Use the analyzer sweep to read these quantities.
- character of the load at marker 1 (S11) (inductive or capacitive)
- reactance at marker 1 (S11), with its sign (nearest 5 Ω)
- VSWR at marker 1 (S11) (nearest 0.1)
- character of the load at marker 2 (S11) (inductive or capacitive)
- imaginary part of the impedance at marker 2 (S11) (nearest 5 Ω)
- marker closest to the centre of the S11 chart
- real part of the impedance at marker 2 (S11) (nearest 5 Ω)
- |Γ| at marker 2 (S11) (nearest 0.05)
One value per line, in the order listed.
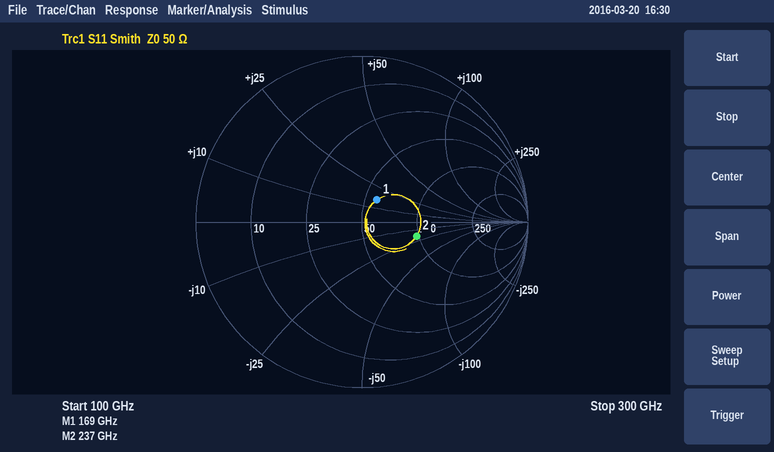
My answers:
inductive
+15 Ω
1.4
capacitive
-20 Ω
marker 1
95 Ω
0.35
